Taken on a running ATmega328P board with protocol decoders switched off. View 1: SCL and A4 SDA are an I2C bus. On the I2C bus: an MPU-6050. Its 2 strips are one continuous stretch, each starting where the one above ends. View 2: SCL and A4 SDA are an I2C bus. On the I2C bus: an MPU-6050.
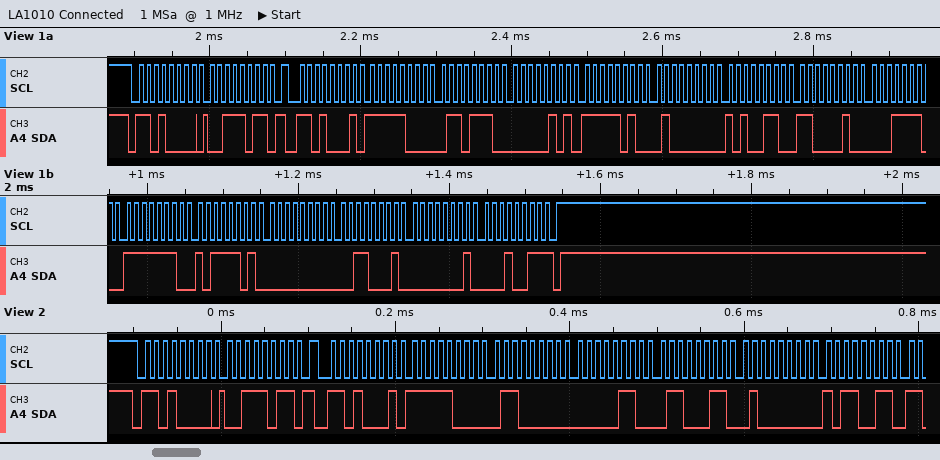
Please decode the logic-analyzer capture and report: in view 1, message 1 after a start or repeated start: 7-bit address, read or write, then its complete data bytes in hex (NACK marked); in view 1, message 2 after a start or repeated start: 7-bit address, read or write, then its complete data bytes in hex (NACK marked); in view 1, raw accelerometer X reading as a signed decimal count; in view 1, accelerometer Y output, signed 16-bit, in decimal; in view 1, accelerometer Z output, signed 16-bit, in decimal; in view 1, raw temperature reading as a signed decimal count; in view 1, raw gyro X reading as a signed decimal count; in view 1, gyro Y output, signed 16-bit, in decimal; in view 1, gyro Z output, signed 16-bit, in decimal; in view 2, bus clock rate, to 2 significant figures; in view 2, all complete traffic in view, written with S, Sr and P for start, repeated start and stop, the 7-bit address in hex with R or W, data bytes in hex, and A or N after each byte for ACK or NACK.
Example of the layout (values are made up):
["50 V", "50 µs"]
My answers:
["0x68 write: 3B", "0x68 read: F8 6E 05 FA 40 A6 C2 1E FE BD 00 31 01 13 NACK", "-1938", "1530", "16550", "-15842", "-323", "49", "275", "100 kHz", "S 68W A 3B A Sr 68R A F8 A 60 A 06 A 63 A 40 A B3 A"]
